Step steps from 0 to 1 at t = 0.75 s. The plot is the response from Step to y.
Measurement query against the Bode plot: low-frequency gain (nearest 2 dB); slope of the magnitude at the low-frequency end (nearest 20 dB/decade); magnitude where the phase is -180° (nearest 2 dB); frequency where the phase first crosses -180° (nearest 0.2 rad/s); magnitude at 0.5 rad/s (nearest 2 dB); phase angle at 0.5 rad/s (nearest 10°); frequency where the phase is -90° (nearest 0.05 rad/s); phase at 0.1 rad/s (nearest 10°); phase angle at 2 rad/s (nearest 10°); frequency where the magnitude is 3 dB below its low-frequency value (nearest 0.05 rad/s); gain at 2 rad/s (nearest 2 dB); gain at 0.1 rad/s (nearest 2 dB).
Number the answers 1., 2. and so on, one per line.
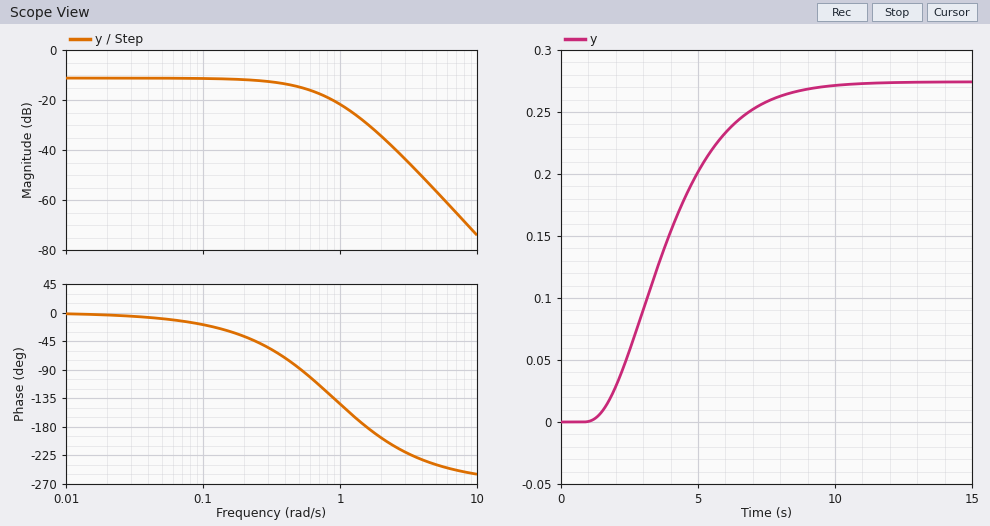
1. -12 dB
2. 0 dB/decade
3. -30 dB
4. 1.6 rad/s
5. -14 dB
6. -90°
7. 0.50 rad/s
8. -20°
9. -200°
10. 0.45 rad/s
11. -34 dB
12. -12 dB
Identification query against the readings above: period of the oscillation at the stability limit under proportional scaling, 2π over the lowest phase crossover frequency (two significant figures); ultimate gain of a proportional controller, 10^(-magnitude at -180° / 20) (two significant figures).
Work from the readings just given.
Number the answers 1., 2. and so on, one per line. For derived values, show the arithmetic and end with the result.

1. 2π / 1.6 = 3.9 s
2. 10^(30 / 20) = 32
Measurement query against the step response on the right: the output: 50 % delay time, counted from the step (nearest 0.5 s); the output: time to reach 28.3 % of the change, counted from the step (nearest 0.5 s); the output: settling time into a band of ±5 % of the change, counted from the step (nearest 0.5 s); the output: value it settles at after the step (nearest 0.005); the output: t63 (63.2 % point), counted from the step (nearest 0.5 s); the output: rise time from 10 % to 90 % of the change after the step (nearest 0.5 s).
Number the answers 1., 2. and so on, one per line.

1. 3.0 s
2. 2.0 s
3. 7.0 s
4. 0.275
5. 3.5 s
6. 4.5 s
